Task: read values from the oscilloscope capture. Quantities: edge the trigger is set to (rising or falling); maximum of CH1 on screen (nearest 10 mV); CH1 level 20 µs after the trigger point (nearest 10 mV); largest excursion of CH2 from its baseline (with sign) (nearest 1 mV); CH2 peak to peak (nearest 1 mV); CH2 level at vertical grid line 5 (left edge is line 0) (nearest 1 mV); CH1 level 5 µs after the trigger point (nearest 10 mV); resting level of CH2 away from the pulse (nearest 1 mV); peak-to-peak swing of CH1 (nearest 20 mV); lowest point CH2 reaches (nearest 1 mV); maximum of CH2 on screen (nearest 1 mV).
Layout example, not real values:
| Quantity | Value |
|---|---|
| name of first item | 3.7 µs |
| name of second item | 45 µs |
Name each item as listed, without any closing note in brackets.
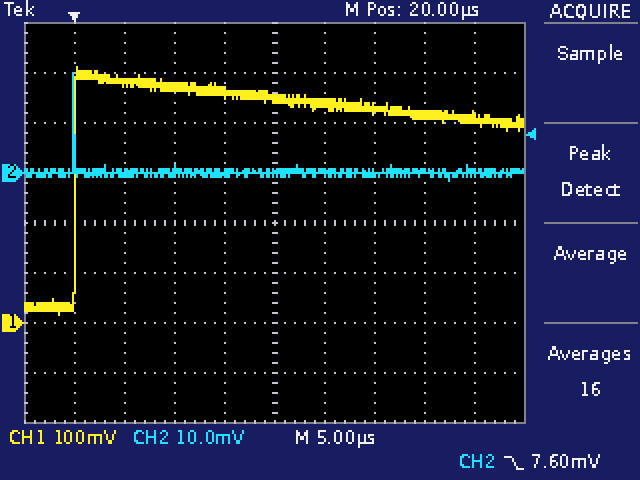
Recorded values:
| Quantity | Value |
|---|---|
| edge the trigger is set to | falling |
| maximum of CH1 on screen | 510 mV |
| CH1 level 20 µs after the trigger point | 450 mV |
| largest excursion of CH2 from its baseline (with sign) | +20 mV |
| CH2 peak to peak | 22 mV |
| CH2 level at vertical grid line 5 (left edge is line 0) | 0 mV |
| CH1 level 5 µs after the trigger point | 480 mV |
| resting level of CH2 away from the pulse | 0 mV |
| peak-to-peak swing of CH1 | 500 mV |
| lowest point CH2 reaches | -2 mV |
| maximum of CH2 on screen | 20 mV |
